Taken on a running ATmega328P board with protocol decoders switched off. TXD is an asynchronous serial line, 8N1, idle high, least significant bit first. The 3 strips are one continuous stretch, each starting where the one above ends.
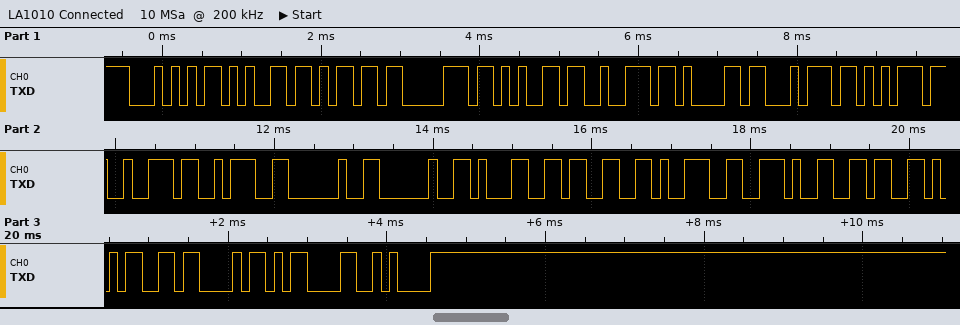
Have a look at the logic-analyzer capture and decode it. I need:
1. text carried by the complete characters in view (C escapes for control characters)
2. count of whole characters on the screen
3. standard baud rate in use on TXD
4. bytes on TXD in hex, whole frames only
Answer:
"Temperatur:  139.65C\r\n"
22
9600 baud
0x54 0x65 0x6D 0x70 0x65 0x72 0x61 0x74 0x75 0x72 0x3A 0x20 0x20 0x31 0x33 0x39 0x2E 0x36 0x35 0x43 0x0D 0x0A
